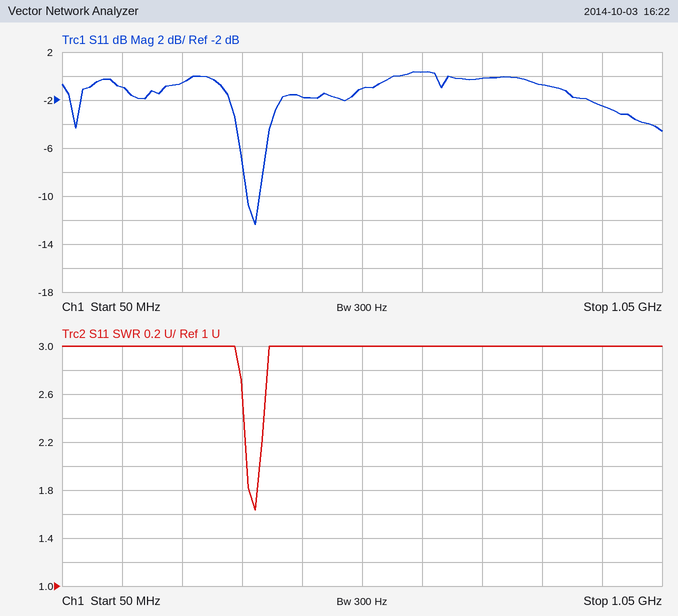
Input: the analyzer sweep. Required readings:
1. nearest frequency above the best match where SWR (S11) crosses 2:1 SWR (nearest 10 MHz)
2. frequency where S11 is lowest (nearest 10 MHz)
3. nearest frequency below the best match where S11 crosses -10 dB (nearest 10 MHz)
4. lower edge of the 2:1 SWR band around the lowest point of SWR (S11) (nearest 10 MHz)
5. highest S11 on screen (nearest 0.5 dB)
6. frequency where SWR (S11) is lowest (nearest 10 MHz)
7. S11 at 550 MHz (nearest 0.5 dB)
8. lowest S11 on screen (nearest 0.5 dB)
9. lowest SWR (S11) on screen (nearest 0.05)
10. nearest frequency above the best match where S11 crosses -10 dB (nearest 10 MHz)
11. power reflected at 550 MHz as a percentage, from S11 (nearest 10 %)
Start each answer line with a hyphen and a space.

- 380 MHz
- 370 MHz
- 360 MHz
- 360 MHz
- 0.5 dB
- 370 MHz
- -1.0 dB
- -12.5 dB
- 1.65
- 380 MHz
- 80 %
